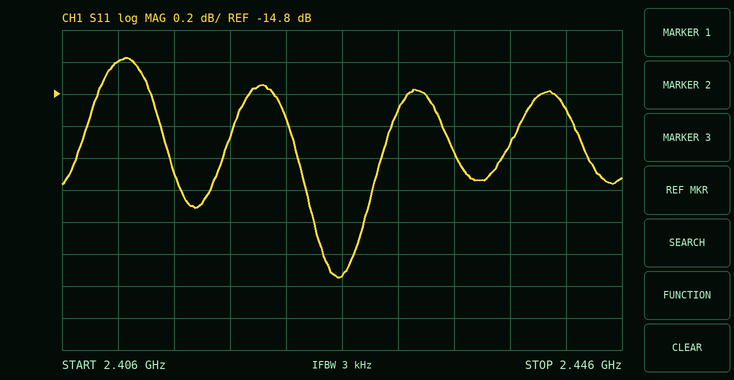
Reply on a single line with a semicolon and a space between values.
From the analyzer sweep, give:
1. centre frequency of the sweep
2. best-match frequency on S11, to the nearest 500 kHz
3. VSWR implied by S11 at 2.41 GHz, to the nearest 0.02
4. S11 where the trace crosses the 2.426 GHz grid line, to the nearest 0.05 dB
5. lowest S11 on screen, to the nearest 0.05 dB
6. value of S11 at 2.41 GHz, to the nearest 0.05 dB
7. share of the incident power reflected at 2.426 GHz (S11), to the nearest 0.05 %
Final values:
2.426 GHz; 2.4255 GHz; 1.46; -15.95 dB; -15.95 dB; -14.60 dB; 2.55 %
